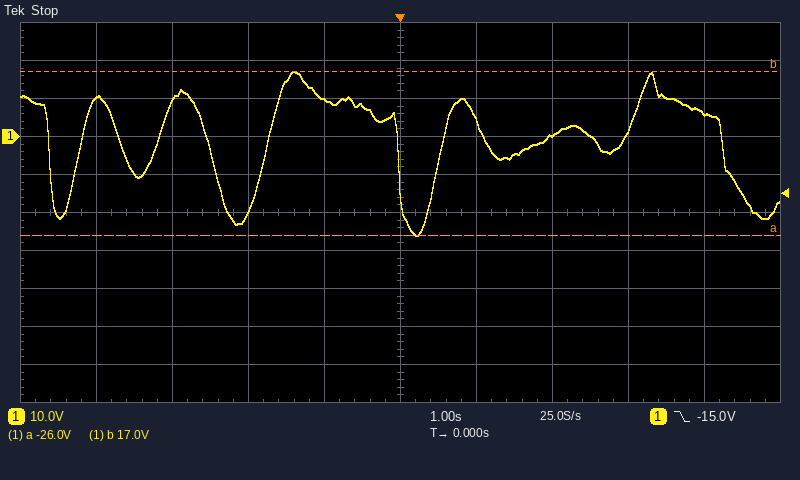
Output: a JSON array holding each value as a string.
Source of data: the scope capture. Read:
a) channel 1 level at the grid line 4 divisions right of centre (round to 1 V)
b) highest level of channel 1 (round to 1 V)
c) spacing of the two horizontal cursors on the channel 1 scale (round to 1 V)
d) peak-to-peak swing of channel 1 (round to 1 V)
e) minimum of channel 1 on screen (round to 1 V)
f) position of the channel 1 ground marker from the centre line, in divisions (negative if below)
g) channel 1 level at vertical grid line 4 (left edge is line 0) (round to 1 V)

["6 V", "17 V", "43 V", "43 V", "-26 V", "+2.0 div", "10 V"]
